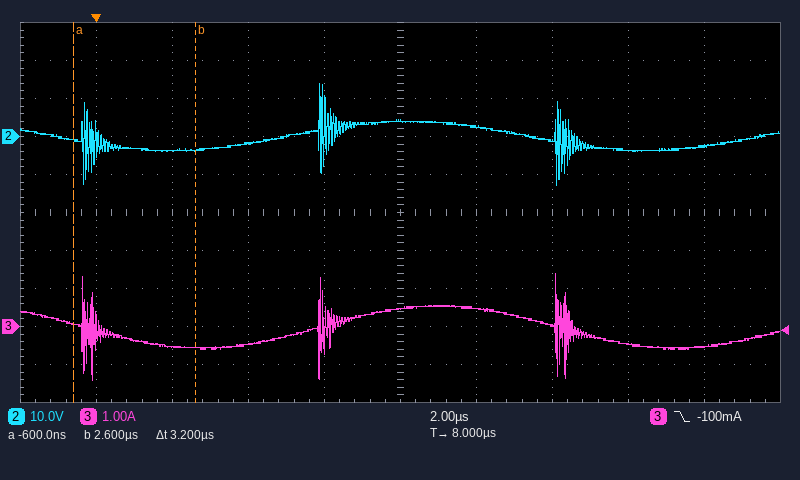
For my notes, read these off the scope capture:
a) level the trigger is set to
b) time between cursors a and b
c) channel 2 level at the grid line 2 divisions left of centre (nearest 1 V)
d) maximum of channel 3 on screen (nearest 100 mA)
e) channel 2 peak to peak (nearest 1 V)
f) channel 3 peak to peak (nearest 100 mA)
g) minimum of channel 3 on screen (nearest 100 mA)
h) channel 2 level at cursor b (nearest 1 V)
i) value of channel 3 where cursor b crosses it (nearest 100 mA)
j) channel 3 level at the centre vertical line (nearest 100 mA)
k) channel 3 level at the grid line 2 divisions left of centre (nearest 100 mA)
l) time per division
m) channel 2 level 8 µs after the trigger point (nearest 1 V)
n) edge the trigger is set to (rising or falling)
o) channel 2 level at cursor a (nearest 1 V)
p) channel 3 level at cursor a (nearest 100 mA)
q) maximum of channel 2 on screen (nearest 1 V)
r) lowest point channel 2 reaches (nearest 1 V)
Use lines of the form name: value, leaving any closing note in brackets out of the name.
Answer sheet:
level the trigger is set to: -100 mA
time between cursors a and b: 3.2 µs
channel 2 level at the grid line 2 divisions left of centre: -2 V
maximum of channel 3 on screen: 1.4 A
channel 2 peak to peak: 27 V
channel 3 peak to peak: 2.8 A
minimum of channel 3 on screen: -1.4 A
channel 2 level at cursor b: -4 V
value of channel 3 where cursor b crosses it: -600 mA
channel 3 level at the centre vertical line: 500 mA
channel 3 level at the grid line 2 divisions left of centre: -500 mA
time per division: 2 µs
channel 2 level 8 µs after the trigger point: 4 V
edge the trigger is set to: falling
channel 2 level at cursor a: -1 V
channel 3 level at cursor a: 100 mA
maximum of channel 2 on screen: 14 V
lowest point channel 2 reaches: -13 V
